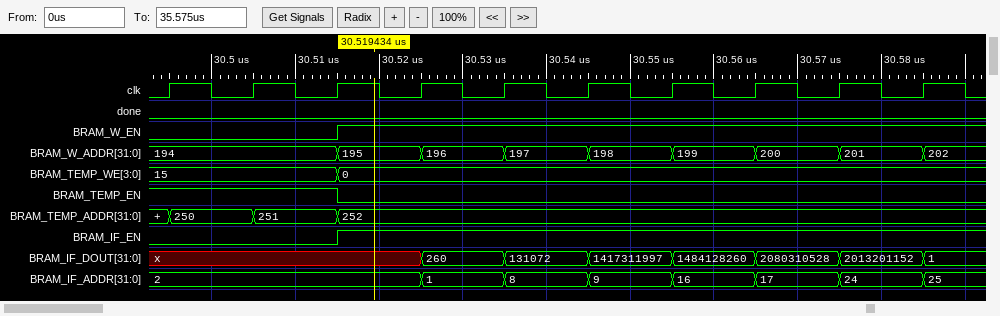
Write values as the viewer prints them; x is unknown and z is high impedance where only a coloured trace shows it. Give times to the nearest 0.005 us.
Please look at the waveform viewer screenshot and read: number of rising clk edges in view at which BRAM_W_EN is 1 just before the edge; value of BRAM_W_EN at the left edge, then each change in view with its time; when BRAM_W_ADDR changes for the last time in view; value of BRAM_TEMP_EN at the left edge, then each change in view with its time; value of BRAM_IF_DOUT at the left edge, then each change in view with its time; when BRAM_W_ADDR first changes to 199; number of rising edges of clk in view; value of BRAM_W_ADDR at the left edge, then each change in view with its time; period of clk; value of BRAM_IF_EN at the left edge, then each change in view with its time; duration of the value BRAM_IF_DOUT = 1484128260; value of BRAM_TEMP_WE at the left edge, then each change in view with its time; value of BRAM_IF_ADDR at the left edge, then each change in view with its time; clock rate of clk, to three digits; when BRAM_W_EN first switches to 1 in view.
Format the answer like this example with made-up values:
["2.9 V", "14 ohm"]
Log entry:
["7", "0, 1 at 30.515 us", "30.585 us", "1, 0 at 30.515 us", "x, 260 at 30.525 us, 131072 at 30.535 us, 1417311997 at 30.545 us, 1484128260 at 30.555 us, 2080310528 at 30.565 us, 2013201152 at 30.575 us, 1 at 30.585 us", "30.555 us", "10", "194, 195 at 30.515 us, 196 at 30.525 us, 197 at 30.535 us, 198 at 30.545 us, 199 at 30.555 us, 200 at 30.565 us, 201 at 30.575 us, 202 at 30.585 us", "0.01 us", "0, 1 at 30.515 us", "0.01 us", "15, 0 at 30.515 us", "2, 1 at 30.525 us, 8 at 30.535 us, 9 at 30.545 us, 16 at 30.555 us, 17 at 30.565 us, 24 at 30.575 us, 25 at 30.585 us", "100 MHz", "30.515 us"]
